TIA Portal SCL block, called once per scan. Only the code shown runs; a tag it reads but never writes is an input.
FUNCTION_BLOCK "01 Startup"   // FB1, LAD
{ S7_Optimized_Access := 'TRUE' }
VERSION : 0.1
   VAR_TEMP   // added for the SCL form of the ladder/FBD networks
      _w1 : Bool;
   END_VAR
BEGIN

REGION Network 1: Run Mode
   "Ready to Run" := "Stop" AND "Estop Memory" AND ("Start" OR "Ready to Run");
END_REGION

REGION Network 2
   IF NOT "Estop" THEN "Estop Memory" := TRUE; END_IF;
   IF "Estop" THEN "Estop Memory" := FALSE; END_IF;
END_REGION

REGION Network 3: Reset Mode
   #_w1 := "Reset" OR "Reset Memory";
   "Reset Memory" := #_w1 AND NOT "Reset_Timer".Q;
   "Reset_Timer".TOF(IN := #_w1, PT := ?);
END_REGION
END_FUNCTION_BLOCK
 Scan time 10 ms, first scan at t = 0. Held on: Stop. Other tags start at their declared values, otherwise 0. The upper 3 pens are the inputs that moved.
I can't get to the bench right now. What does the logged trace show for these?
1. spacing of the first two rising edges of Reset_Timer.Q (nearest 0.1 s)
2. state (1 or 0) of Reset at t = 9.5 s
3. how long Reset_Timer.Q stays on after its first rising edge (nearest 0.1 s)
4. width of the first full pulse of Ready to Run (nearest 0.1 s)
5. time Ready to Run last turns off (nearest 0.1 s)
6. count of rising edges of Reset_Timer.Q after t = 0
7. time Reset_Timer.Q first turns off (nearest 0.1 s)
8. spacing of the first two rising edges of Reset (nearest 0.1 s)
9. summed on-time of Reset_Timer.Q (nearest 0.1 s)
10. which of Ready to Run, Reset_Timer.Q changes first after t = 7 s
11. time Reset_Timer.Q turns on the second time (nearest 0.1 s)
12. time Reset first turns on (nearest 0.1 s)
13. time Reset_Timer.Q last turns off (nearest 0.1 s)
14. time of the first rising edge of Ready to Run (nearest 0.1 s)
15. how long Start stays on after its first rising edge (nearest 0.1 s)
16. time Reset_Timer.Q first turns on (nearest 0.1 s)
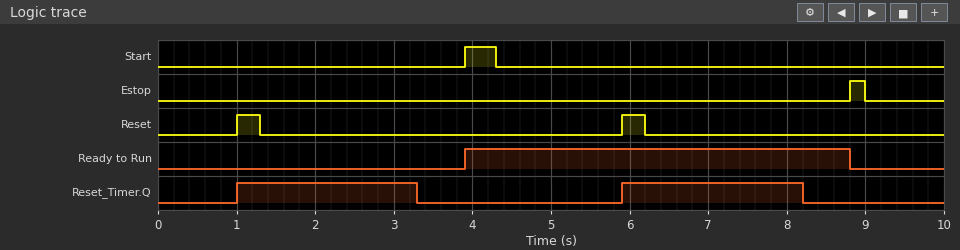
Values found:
4.9 s
0
2.3 s
4.9 s
8.8 s
2
3.3 s
4.9 s
4.6 s
Reset_Timer.Q
5.9 s
1.0 s
8.2 s
3.9 s
0.4 s
1.0 s
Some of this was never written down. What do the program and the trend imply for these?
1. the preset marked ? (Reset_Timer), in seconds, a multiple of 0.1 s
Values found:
2.0 s
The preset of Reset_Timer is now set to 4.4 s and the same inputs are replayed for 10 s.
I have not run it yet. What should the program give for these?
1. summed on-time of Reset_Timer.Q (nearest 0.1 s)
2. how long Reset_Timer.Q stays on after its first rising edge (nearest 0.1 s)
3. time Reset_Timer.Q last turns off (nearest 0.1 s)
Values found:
8.8 s
4.7 s
5.7 s
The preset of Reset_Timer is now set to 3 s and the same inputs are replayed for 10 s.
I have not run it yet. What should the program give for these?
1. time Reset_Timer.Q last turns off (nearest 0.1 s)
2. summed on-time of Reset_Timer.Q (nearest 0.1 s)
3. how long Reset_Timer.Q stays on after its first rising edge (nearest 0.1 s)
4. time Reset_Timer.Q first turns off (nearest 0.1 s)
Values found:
9.2 s
6.6 s
3.3 s
4.3 s
